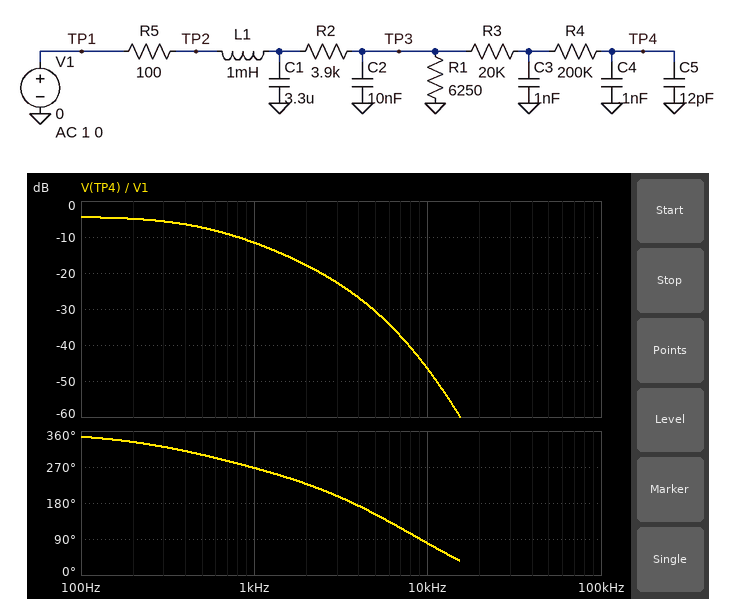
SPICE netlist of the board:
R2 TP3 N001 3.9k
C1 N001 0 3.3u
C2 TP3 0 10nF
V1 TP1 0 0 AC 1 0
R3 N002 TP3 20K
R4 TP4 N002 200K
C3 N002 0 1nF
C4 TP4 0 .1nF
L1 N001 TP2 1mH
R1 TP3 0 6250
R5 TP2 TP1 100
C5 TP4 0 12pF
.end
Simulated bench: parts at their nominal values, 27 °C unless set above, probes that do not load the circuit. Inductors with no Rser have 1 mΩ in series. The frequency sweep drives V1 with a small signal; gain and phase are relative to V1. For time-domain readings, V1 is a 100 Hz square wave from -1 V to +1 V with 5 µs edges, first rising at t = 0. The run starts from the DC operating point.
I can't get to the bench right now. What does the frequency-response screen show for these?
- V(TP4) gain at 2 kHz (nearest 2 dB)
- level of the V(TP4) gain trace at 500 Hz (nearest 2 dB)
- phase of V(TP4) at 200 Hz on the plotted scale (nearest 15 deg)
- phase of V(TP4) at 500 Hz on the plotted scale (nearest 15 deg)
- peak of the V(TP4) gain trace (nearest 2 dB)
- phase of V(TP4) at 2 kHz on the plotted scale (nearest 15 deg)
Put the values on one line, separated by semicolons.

-18 dB; -8 dB; 330 deg; 300 deg; -4 dB; 225 deg
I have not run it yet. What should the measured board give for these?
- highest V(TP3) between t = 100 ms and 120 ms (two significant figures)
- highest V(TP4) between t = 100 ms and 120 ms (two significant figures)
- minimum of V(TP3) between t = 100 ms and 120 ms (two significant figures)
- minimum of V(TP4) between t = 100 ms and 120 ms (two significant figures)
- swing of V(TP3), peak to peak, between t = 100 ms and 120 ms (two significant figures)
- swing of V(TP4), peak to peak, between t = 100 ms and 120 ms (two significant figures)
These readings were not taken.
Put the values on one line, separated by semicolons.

610 mV; 610 mV; -610 mV; -610 mV; 1.2 V; 1.2 V
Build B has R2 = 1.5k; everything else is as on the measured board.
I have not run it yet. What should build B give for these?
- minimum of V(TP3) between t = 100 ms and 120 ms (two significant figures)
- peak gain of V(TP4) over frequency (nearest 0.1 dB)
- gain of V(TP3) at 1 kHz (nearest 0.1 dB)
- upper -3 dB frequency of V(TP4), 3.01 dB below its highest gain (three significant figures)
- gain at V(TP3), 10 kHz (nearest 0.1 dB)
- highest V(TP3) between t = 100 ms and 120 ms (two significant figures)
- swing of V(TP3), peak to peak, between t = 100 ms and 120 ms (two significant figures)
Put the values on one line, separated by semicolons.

-800 mV; -2.0 dB; -9.0 dB; 496 Hz; -31.8 dB; 800 mV; 1.6 V
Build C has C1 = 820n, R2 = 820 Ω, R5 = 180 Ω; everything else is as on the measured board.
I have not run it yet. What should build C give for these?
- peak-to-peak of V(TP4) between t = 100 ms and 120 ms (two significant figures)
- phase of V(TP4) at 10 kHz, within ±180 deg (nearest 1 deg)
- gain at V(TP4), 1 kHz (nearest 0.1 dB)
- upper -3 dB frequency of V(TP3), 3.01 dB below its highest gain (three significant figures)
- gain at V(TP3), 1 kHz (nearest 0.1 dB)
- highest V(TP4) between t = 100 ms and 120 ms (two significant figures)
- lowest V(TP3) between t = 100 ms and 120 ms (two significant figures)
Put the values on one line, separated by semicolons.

1.7 V; 127 deg; -4.0 dB; 1.13 kHz; -3.8 dB; 860 mV; -860 mV
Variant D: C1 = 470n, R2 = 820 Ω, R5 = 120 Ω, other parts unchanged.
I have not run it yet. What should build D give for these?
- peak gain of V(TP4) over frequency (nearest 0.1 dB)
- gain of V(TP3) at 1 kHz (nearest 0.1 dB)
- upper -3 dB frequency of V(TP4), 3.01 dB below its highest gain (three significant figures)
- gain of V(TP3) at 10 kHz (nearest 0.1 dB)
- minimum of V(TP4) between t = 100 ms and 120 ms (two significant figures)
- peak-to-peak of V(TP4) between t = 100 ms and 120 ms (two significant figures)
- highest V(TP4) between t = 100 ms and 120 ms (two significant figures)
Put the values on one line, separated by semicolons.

-1.2 dB; -1.6 dB; 2.43 kHz; -13.5 dB; -870 mV; 1.7 V; 870 mV
